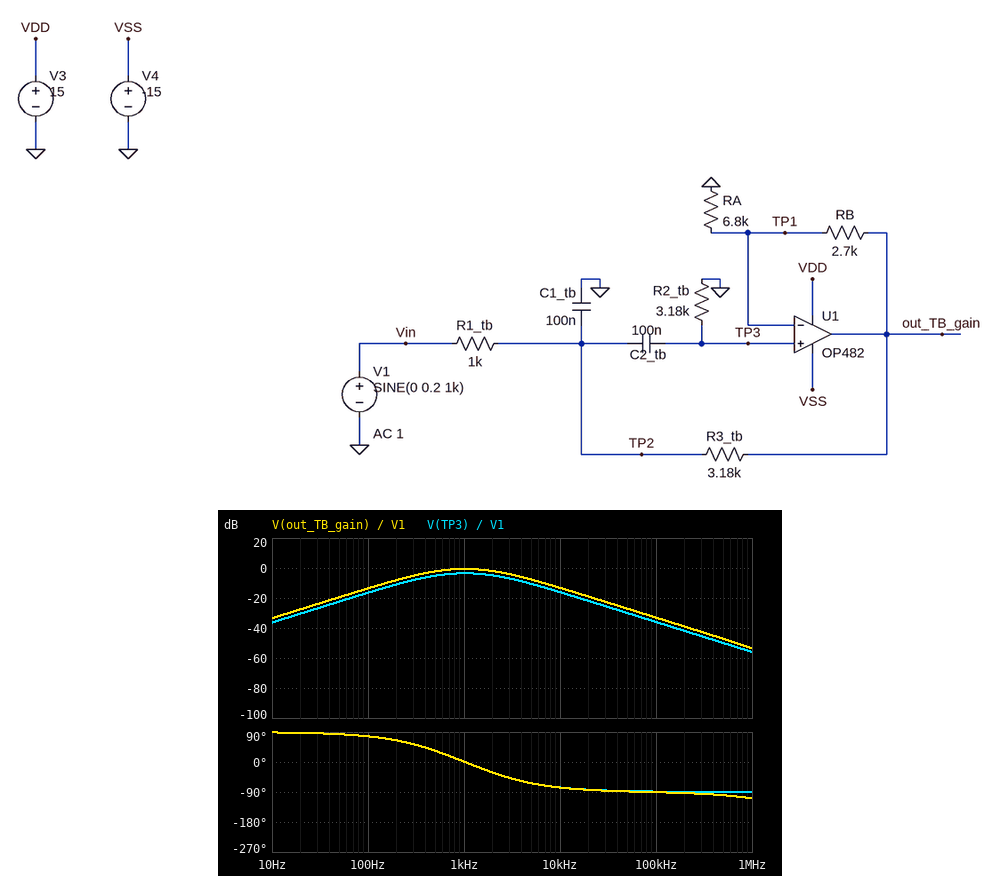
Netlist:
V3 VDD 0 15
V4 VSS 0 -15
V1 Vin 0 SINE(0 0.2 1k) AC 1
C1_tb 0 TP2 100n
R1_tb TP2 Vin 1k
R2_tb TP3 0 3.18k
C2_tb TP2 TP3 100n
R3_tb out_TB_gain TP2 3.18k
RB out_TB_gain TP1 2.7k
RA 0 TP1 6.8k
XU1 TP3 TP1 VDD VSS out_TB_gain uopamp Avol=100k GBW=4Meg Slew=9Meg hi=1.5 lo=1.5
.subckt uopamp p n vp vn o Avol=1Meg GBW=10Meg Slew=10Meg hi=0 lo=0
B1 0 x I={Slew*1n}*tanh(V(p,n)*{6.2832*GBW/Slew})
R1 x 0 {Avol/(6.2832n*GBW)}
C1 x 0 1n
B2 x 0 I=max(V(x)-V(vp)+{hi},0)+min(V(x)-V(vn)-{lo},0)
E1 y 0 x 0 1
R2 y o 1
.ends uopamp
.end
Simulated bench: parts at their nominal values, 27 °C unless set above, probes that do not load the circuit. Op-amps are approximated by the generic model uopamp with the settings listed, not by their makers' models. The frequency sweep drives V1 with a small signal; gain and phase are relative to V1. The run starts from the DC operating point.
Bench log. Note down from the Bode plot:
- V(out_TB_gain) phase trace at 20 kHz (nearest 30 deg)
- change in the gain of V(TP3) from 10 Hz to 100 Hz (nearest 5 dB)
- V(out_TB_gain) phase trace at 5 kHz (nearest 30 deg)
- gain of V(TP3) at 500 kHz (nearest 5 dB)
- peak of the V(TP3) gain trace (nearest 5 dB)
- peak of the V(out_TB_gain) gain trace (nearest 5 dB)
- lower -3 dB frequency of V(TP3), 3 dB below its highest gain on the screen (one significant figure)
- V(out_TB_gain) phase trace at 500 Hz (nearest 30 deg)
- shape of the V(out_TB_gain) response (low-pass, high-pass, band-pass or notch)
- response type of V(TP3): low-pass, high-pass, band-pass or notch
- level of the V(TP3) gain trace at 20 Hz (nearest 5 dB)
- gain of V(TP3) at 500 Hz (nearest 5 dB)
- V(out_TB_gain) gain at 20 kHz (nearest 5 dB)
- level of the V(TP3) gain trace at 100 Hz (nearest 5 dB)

-90 deg
20 dB
-60 deg
-50 dB
-5 dB
0 dB
400 Hz
30 deg
band-pass
band-pass
-30 dB
-5 dB
-20 dB
-15 dB
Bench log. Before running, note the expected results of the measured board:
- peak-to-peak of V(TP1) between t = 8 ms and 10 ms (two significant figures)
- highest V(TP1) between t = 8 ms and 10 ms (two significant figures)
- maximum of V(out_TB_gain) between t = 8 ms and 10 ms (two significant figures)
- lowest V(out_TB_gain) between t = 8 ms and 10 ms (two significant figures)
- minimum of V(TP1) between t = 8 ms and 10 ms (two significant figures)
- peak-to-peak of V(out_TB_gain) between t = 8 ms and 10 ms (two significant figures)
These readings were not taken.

270 mV
130 mV
190 mV
-190 mV
-130 mV
370 mV
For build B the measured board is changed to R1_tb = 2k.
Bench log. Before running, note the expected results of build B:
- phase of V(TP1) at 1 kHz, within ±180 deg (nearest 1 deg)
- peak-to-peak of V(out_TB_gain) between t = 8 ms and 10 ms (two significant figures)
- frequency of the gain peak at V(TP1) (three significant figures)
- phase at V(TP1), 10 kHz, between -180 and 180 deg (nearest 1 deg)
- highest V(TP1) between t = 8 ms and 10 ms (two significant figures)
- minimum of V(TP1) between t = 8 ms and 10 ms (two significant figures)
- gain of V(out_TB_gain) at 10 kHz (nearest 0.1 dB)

-12 deg
270 mV
805 Hz
-81 deg
97 mV
-97 mV
-19.1 dB
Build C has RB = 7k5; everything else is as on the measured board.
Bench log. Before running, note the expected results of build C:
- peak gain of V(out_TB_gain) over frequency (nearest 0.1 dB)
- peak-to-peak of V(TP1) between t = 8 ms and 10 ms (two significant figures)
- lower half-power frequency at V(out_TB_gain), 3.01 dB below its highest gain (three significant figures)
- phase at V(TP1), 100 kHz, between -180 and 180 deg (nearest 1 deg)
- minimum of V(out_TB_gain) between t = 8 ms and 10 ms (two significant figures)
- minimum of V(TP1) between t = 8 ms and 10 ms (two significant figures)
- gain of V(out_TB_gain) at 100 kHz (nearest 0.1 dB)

4.3 dB
310 mV
425 Hz
-92 deg
-330 mV
-160 mV
-29.5 dB
